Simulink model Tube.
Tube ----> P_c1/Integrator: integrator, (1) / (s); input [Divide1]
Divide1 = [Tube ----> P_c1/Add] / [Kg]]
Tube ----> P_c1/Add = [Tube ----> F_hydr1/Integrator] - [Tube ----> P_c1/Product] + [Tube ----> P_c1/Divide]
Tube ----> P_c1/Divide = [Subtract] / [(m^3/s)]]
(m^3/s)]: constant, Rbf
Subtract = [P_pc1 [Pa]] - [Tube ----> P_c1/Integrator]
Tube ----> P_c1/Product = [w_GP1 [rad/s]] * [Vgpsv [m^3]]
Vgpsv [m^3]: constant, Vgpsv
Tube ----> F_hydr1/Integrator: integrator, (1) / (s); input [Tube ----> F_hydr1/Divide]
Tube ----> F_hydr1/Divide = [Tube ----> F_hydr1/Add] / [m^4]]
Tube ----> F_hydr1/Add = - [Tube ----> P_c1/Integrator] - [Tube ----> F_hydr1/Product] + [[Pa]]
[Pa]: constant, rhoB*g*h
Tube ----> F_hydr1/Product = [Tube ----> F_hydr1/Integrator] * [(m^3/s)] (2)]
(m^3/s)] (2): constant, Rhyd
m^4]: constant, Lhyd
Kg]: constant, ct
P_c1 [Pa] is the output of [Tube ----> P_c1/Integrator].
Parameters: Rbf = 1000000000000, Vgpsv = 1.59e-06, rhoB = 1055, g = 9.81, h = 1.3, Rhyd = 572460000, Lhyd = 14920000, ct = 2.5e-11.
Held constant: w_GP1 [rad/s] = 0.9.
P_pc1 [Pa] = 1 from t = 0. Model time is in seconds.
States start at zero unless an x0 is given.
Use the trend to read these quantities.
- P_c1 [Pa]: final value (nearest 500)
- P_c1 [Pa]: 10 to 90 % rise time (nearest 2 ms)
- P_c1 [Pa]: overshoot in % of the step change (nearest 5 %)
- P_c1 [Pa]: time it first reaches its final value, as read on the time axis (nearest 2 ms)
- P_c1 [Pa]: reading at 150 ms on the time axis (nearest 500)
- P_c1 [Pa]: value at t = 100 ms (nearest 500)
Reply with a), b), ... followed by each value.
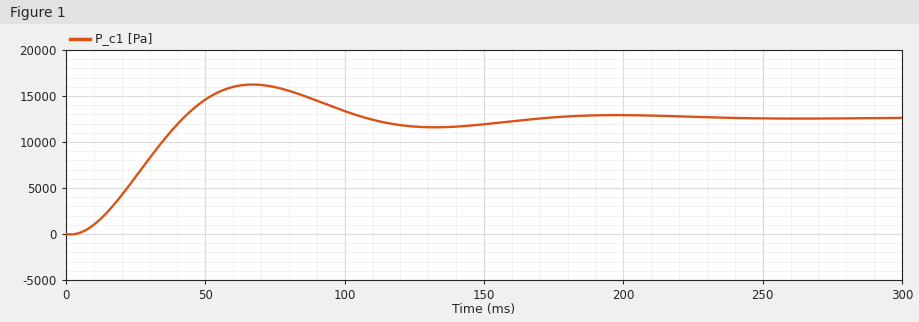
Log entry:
a) 12500
b) 28 ms
c) 30 %
d) 42 ms
e) 12000
f) 13500
